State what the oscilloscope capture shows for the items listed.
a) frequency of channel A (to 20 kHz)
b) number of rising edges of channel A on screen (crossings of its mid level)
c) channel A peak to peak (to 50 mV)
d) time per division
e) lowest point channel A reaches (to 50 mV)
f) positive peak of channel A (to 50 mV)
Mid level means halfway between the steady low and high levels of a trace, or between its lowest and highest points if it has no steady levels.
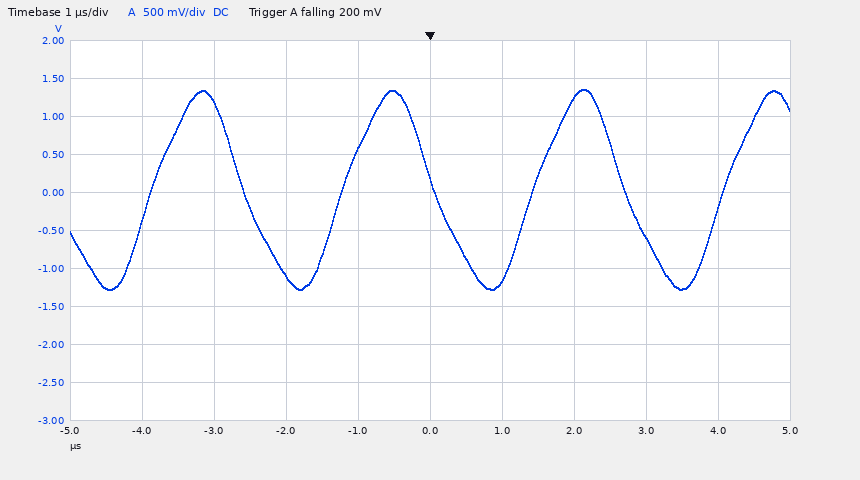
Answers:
380 kHz
4
2.65 V
1 µs
-1.30 V
1.35 V
